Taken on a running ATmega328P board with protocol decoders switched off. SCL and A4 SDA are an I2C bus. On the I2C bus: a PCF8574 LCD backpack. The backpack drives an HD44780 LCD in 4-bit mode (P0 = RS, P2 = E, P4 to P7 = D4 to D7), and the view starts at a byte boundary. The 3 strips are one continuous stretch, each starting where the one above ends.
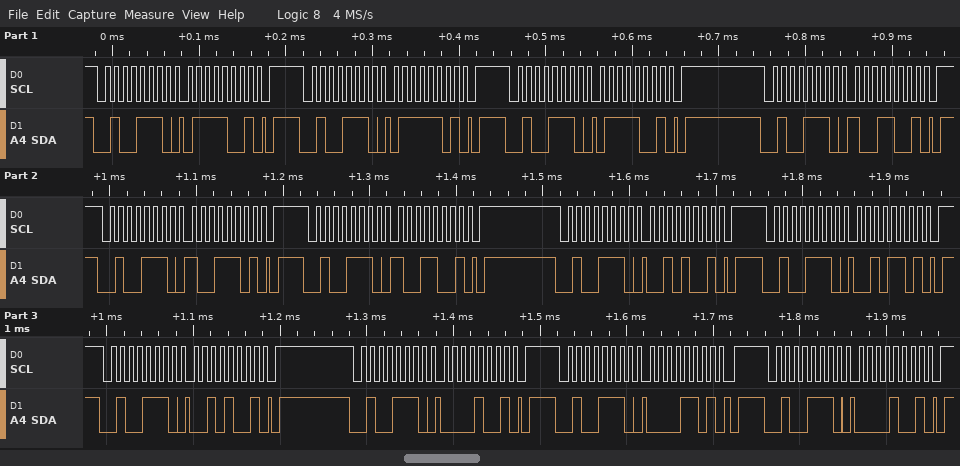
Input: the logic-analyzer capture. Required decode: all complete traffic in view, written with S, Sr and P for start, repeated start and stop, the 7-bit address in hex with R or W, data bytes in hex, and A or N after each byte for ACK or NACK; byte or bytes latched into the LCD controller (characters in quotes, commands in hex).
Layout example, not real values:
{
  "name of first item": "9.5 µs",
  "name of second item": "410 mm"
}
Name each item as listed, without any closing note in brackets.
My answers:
{
  "all complete traffic in view, written with S, Sr and P for start, repeated start and stop, the 7-bit address in hex with R or W, data bytes in hex, and A or N after each byte for ACK or NACK": "S 27W A 79 A P S 27W A 7D A P S 27W A 79 A P S 27W A 99 A P S 27W A 9D A P S 27W A 99 A P S 27W A 29 A P S 27W A 2D A P S 27W A 29 A P S 27W A 09 A P S 27W A 0D A P S 27W A 09 A P",
  "byte or bytes latched into the LCD controller": "'y' ' '"
}
